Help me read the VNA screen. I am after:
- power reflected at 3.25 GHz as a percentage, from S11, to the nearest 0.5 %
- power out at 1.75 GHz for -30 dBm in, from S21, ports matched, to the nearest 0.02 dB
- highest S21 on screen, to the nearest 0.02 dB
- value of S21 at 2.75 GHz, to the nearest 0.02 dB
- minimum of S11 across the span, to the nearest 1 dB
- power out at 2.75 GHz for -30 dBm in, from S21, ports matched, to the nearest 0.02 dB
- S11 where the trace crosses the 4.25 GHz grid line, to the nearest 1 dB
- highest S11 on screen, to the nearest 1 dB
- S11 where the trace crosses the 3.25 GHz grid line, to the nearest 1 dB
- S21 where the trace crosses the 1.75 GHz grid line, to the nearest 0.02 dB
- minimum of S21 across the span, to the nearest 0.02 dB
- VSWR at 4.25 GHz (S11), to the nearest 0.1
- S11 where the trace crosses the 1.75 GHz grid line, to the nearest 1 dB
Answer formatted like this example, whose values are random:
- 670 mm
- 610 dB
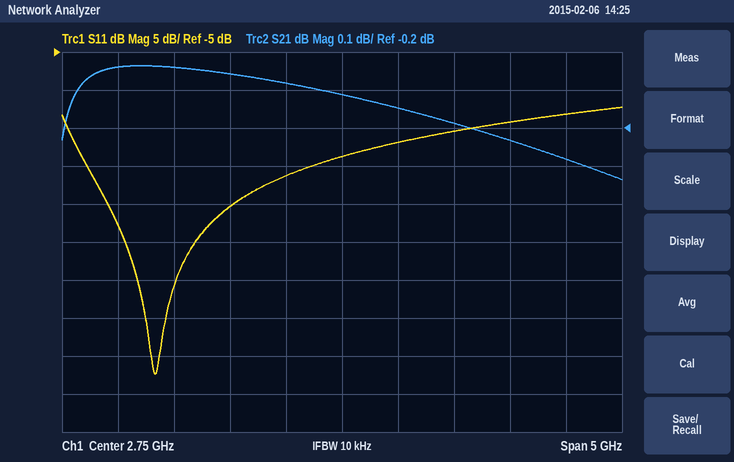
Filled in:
- 2.0 %
- -30.06 dBm
- -0.04 dB
- -0.12 dB
- -47 dB
- -30.12 dBm
- -14 dB
- -12 dB
- -17 dB
- -0.06 dB
- -0.34 dB
- 1.5
- -25 dB
